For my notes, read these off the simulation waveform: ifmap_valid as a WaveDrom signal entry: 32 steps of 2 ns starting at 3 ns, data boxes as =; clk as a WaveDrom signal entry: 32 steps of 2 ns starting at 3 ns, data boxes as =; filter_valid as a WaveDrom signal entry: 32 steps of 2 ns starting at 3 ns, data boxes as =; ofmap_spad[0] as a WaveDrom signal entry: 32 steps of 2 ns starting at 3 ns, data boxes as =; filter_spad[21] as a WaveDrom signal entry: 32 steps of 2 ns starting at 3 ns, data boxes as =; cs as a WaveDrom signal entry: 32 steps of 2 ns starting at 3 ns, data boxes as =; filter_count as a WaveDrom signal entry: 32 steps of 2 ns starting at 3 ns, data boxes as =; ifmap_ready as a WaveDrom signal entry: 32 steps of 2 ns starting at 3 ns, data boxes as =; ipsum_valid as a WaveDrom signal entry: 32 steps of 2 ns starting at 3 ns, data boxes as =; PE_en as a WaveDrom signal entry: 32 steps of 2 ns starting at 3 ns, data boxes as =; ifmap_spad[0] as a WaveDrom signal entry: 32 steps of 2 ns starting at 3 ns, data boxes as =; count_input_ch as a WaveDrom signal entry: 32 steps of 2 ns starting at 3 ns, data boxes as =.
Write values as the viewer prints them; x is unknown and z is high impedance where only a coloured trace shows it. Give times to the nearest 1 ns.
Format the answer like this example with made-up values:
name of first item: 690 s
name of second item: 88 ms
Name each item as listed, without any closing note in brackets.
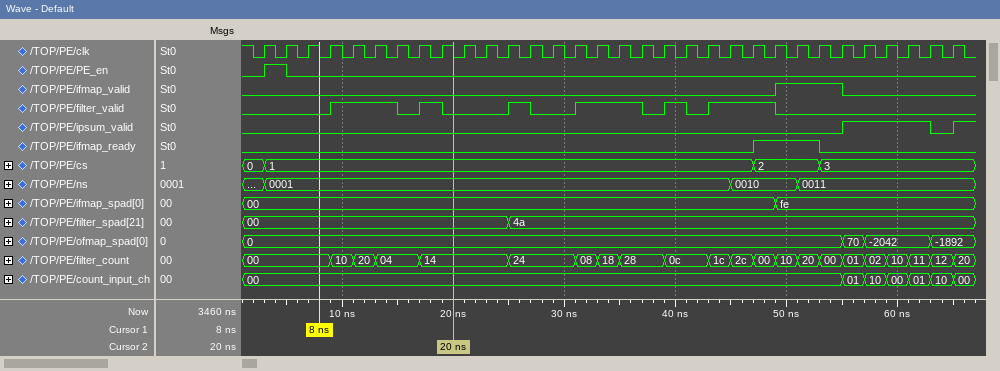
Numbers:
ifmap_valid as a WaveDrom signal entry: 32 steps of 2 ns starting at 3 ns, data boxes as =: {name: 'ifmap_valid', wave: '0......................1..0.....'}
clk as a WaveDrom signal entry: 32 steps of 2 ns starting at 3 ns, data boxes as =: {name: 'clk', wave: 'p...............................'}
filter_valid as a WaveDrom signal entry: 32 steps of 2 ns starting at 3 ns, data boxes as =: {name: 'filter_valid', wave: '0..1..010..10.1..0101..0........'}
ofmap_spad[0] as a WaveDrom signal entry: 32 steps of 2 ns starting at 3 ns, data boxes as =: {name: 'ofmap_spad[0]', wave: '=.........................==..=.', data: '0 70 -2042 -1892'}
filter_spad[21] as a WaveDrom signal entry: 32 steps of 2 ns starting at 3 ns, data boxes as =: {name: 'filter_spad[21]', wave: '=..........=....................', data: '00 4a'}
cs as a WaveDrom signal entry: 32 steps of 2 ns starting at 3 ns, data boxes as =: {name: 'cs', wave: '=.....................=..=......', data: '1 2 3'}
filter_count as a WaveDrom signal entry: 32 steps of 2 ns starting at 3 ns, data boxes as =: {name: 'filter_count', wave: '=..===.=...=..===.=.============', data: '00 10 20 04 14 24 08 18 28 0c 1c 2c 00 10 20 00 01 02 10 11 12 20'}
ifmap_ready as a WaveDrom signal entry: 32 steps of 2 ns starting at 3 ns, data boxes as =: {name: 'ifmap_ready', wave: '0.....................1..0......'}
ipsum_valid as a WaveDrom signal entry: 32 steps of 2 ns starting at 3 ns, data boxes as =: {name: 'ipsum_valid', wave: '0.........................1...01'}
PE_en as a WaveDrom signal entry: 32 steps of 2 ns starting at 3 ns, data boxes as =: {name: 'PE_en', wave: '10..............................'}
ifmap_spad[0] as a WaveDrom signal entry: 32 steps of 2 ns starting at 3 ns, data boxes as =: {name: 'ifmap_spad[0]', wave: '=......................=........', data: '00 fe'}
count_input_ch as a WaveDrom signal entry: 32 steps of 2 ns starting at 3 ns, data boxes as =: {name: 'count_input_ch', wave: '=.........................======', data: '00 01 10 00 01 10 00'}
